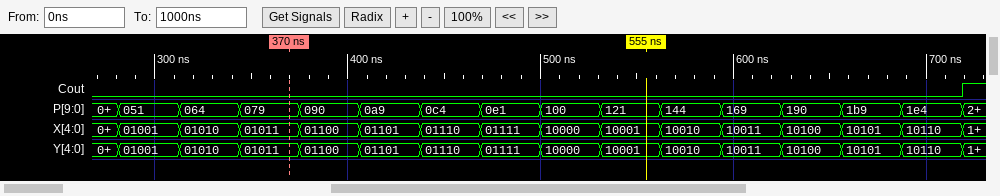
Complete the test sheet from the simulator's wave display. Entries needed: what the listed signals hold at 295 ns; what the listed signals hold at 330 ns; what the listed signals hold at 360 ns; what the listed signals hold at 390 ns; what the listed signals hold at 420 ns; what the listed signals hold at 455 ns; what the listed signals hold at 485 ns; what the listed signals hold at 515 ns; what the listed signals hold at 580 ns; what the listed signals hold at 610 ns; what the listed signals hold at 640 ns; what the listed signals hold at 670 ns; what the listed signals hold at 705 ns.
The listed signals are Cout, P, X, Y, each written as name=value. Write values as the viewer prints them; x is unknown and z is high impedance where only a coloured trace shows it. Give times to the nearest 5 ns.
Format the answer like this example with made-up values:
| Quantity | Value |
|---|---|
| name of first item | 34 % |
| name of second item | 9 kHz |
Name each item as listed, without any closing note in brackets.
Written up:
| Quantity | Value |
|---|---|
| what the listed signals hold at 295 ns | Cout=0, P=051, X=01001, Y=01001 |
| what the listed signals hold at 330 ns | Cout=0, P=064, X=01010, Y=01010 |
| what the listed signals hold at 360 ns | Cout=0, P=079, X=01011, Y=01011 |
| what the listed signals hold at 390 ns | Cout=0, P=090, X=01100, Y=01100 |
| what the listed signals hold at 420 ns | Cout=0, P=0a9, X=01101, Y=01101 |
| what the listed signals hold at 455 ns | Cout=0, P=0c4, X=01110, Y=01110 |
| what the listed signals hold at 485 ns | Cout=0, P=0e1, X=01111, Y=01111 |
| what the listed signals hold at 515 ns | Cout=0, P=100, X=10000, Y=10000 |
| what the listed signals hold at 580 ns | Cout=0, P=144, X=10010, Y=10010 |
| what the listed signals hold at 610 ns | Cout=0, P=169, X=10011, Y=10011 |
| what the listed signals hold at 640 ns | Cout=0, P=190, X=10100, Y=10100 |
| what the listed signals hold at 670 ns | Cout=0, P=1b9, X=10101, Y=10101 |
| what the listed signals hold at 705 ns | Cout=0, P=1e4, X=10110, Y=10110 |
